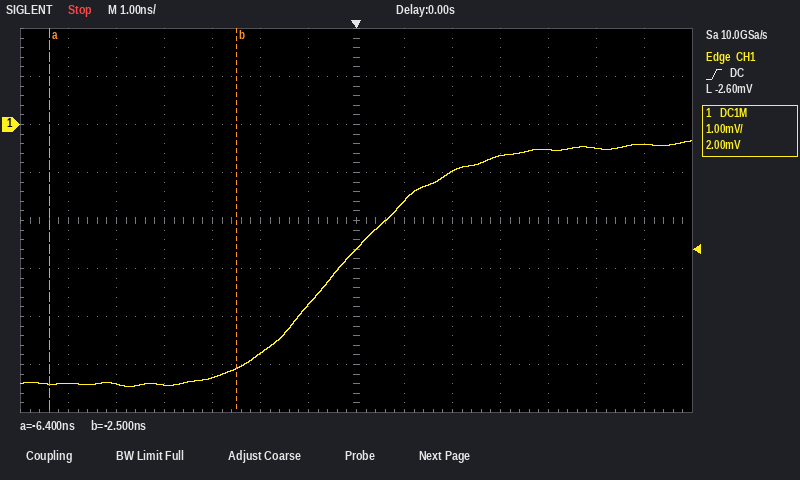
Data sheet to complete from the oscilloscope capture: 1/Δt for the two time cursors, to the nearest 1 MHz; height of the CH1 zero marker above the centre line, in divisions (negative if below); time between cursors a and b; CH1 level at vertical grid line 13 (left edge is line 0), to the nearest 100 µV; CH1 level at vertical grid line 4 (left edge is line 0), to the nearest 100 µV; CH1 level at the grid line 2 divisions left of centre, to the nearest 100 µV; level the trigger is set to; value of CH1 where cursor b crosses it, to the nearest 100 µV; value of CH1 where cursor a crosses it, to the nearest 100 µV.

256 MHz
+2.0 div
3.9 ns
-400 µV
-5.3 mV
-4.8 mV
-2.60 mV
-5.1 mV
-5.4 mV
